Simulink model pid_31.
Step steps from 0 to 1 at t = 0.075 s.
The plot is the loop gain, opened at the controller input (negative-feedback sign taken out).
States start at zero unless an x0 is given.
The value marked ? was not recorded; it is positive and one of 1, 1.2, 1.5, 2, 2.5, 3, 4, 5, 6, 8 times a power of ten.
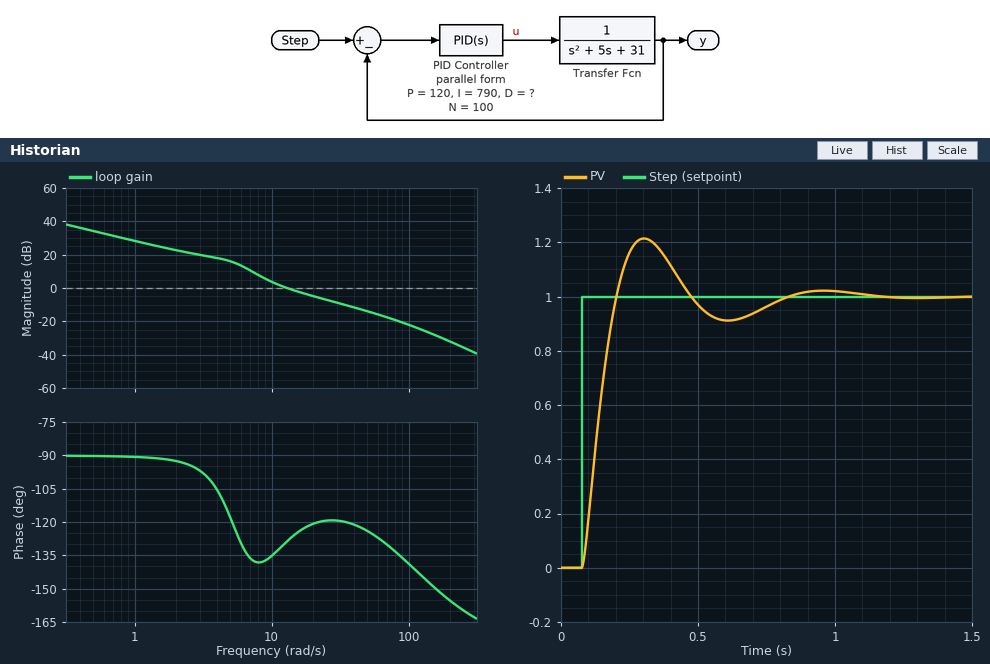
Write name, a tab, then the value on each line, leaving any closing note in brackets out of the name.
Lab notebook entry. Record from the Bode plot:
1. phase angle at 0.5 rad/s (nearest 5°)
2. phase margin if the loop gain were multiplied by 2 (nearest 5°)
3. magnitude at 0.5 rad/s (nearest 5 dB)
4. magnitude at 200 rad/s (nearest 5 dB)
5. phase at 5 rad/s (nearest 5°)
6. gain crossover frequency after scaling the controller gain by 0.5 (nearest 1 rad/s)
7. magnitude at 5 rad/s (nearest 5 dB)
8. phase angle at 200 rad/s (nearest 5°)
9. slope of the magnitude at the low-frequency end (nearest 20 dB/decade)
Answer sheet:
phase angle at 0.5 rad/s	-90°
phase margin if the loop gain were multiplied by 2	60°
magnitude at 0.5 rad/s	35 dB
magnitude at 200 rad/s	-30 dB
phase at 5 rad/s	-120°
gain crossover frequency after scaling the controller gain by 0.5	9 rad/s
magnitude at 5 rad/s	15 dB
phase angle at 200 rad/s	-155°
slope of the magnitude at the low-frequency end	-20 dB/decade
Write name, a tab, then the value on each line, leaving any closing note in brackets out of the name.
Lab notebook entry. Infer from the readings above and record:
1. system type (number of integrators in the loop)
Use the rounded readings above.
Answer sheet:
system type	1
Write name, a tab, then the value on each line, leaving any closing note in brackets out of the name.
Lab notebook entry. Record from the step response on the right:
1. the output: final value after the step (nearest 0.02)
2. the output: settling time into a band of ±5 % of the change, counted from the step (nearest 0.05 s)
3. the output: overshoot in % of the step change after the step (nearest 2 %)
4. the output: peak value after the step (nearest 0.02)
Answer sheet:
the output: final value after the step	1.00
the output: settling time into a band of ±5 % of the change, counted from the step	0.65 s
the output: overshoot in % of the step change after the step	22 %
the output: peak value after the step	1.22
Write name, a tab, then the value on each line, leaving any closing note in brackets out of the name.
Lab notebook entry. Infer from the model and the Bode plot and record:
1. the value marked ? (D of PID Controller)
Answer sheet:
the value marked ?	10
